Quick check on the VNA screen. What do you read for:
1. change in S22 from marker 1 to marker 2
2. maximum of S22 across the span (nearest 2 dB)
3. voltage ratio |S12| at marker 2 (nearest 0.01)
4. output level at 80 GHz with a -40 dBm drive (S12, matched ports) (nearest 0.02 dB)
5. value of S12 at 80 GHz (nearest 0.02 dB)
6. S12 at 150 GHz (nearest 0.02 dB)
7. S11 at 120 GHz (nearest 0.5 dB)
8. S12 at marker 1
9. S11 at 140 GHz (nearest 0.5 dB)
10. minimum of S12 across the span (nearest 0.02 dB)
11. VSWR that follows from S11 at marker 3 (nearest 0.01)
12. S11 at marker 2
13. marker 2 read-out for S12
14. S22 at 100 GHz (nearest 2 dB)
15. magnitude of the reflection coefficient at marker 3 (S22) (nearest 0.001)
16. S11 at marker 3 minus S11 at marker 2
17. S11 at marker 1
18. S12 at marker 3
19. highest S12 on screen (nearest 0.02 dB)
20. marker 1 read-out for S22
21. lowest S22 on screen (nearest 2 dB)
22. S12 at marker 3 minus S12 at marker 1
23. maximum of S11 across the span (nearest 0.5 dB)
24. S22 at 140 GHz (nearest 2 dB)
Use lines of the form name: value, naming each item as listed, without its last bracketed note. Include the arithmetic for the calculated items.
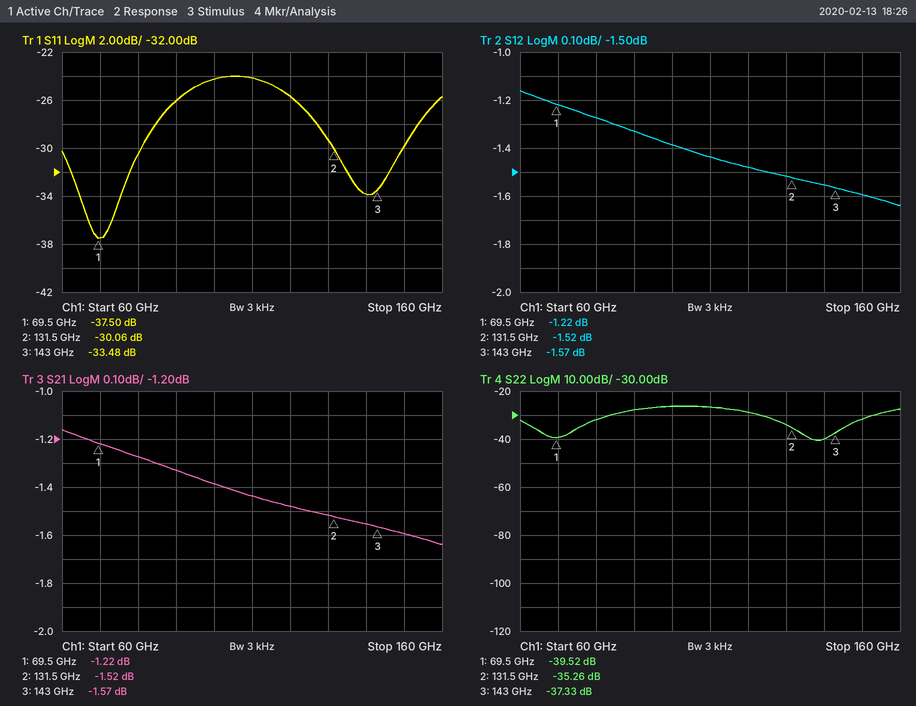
change in S22 from marker 1 to marker 2: -35.26 − (-39.52) = 4.26 dB
maximum of S22 across the span: -26 dB
voltage ratio |S12| at marker 2: 10^(-1.52/20) ≈ 0.84
output level at 80 GHz with a -40 dBm drive (S12, matched ports): -40 dBm + (-1.28 dB) = -41.28 dBm
value of S12 at 80 GHz: -1.28 dB
S12 at 150 GHz: -1.60 dB
S11 at 120 GHz: -25.5 dB
S12 at marker 1: -1.22 dB
S11 at 140 GHz: -34.0 dB
minimum of S12 across the span: -1.64 dB
VSWR that follows from S11 at marker 3: (1 + 0.0212)/(1 − 0.0212) ≈ 1.04
S11 at marker 2: -30.06 dB
marker 2 read-out for S12: -1.52 dB
S22 at 100 GHz: -26 dB
magnitude of the reflection coefficient at marker 3 (S22): 10^(-37.33/20) ≈ 0.014
S11 at marker 3 minus S11 at marker 2: -33.48 − (-30.06) = -3.42 dB
S11 at marker 1: -37.50 dB
S12 at marker 3: -1.57 dB
highest S12 on screen: -1.16 dB
marker 1 read-out for S22: -39.52 dB
lowest S22 on screen: -40 dB
S12 at marker 3 minus S12 at marker 1: -1.57 − (-1.22) = -0.35 dB
maximum of S11 across the span: -24.0 dB
S22 at 140 GHz: -40 dB
